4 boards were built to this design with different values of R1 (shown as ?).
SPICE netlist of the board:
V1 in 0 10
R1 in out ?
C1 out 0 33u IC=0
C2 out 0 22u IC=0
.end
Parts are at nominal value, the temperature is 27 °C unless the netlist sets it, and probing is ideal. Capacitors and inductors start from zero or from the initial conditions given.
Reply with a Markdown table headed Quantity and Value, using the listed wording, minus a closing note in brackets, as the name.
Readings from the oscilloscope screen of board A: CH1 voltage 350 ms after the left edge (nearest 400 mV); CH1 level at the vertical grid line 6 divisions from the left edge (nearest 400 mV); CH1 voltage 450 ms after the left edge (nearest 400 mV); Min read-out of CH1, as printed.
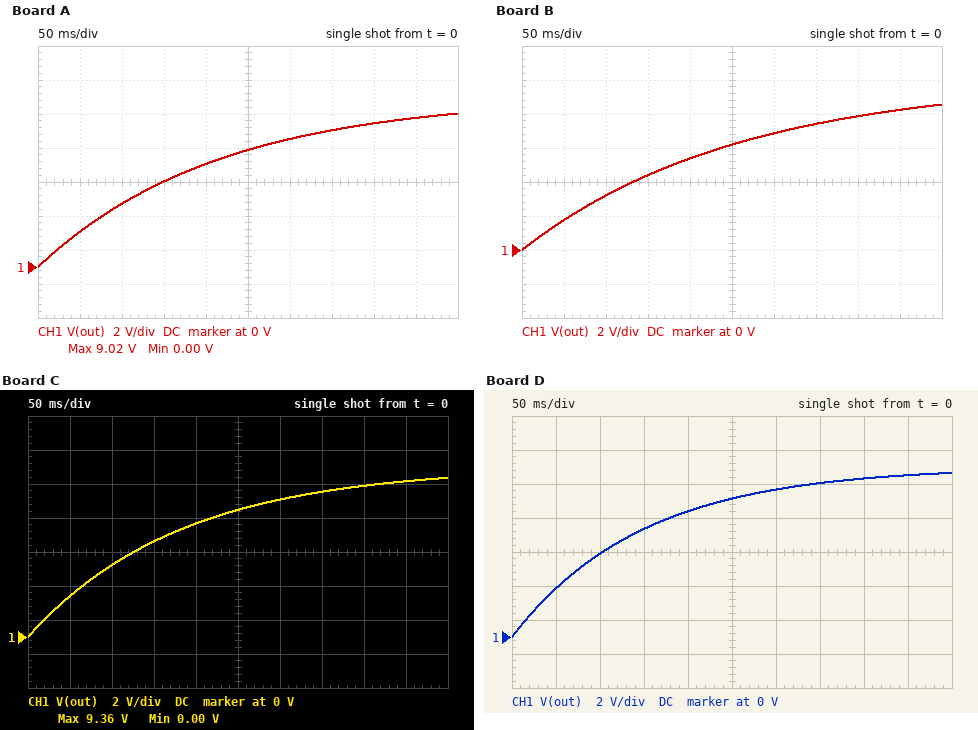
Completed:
| Quantity | Value |
|---|---|
| CH1 voltage 350 ms after the left edge | 8.0 V |
| CH1 level at the vertical grid line 6 divisions from the left edge | 7.6 V |
| CH1 voltage 450 ms after the left edge | 8.8 V |
| Min read-out of CH1, as printed | 0.00 V |
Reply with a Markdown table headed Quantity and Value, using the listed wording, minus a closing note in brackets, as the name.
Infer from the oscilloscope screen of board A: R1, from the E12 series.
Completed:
| Quantity | Value |
|---|---|
| R1, from the E12 series | 3.9 kΩ |
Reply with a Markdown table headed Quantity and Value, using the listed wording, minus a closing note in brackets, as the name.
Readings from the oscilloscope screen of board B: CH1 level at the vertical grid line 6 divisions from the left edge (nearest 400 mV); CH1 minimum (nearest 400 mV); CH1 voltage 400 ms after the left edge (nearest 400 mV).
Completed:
| Quantity | Value |
|---|---|
| CH1 level at the vertical grid line 6 divisions from the left edge | 6.8 V |
| CH1 minimum | 0 V |
| CH1 voltage 400 ms after the left edge | 8.0 V |
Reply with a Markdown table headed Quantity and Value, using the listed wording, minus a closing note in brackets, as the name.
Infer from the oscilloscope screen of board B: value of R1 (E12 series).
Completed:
| Quantity | Value |
|---|---|
| value of R1 | 4.7 kΩ |
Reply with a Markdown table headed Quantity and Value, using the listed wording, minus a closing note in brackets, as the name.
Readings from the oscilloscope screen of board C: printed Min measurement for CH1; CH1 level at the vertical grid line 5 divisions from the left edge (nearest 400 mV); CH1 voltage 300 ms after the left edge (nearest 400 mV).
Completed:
| Quantity | Value |
|---|---|
| printed Min measurement for CH1 | 0.00 V |
| CH1 level at the vertical grid line 5 divisions from the left edge | 7.6 V |
| CH1 voltage 300 ms after the left edge | 8.0 V |
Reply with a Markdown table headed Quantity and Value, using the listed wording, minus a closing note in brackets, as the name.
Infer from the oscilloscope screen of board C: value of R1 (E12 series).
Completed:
| Quantity | Value |
|---|---|
| value of R1 | 3.3 kΩ |
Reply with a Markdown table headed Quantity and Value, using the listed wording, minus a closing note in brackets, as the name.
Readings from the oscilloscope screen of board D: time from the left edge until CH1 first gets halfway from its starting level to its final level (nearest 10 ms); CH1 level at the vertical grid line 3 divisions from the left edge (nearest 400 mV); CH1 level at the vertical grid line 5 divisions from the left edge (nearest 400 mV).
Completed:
| Quantity | Value |
|---|---|
| time from the left edge until CH1 first gets halfway from its starting level to its final level | 100 ms |
| CH1 level at the vertical grid line 3 divisions from the left edge | 6.4 V |
| CH1 level at the vertical grid line 5 divisions from the left edge | 8.0 V |
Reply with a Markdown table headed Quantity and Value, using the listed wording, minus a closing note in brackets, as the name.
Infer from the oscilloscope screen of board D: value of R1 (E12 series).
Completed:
| Quantity | Value |
|---|---|
| value of R1 | 2.7 kΩ |
